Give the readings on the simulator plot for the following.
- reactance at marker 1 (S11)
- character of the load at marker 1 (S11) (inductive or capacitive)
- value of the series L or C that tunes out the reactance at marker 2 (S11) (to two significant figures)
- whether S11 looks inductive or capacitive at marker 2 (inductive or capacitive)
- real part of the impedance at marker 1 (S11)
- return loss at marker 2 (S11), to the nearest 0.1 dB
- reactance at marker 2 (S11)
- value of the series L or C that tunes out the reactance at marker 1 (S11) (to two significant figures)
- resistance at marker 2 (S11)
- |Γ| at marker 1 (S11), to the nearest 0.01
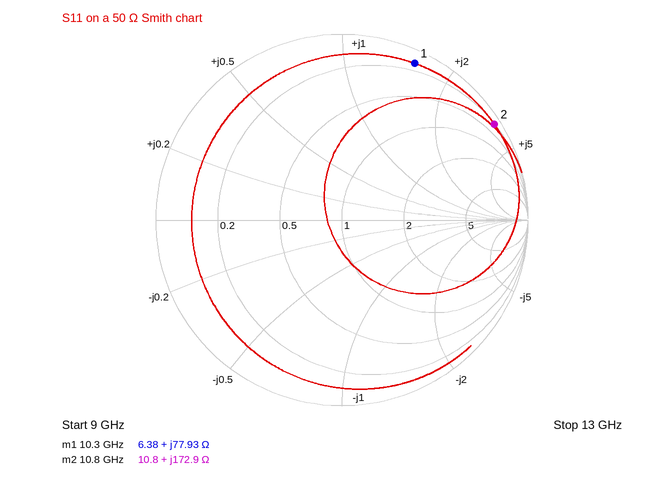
+77.93 Ω
inductive
85 fF
inductive
6.38 Ω
0.3 dB
+172.9 Ω
200 fF
10.8 Ω
0.93
